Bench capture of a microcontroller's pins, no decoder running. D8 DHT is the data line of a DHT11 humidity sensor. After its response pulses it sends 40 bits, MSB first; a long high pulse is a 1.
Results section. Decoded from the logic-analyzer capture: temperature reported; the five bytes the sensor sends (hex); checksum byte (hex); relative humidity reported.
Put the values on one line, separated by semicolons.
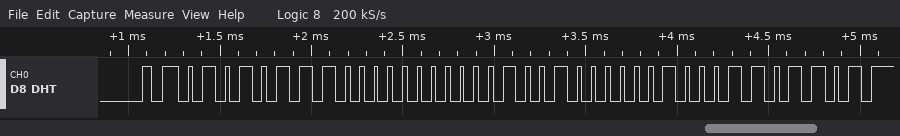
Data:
18.4 °C; 57 00 12 04 6D; 0x6D; 87 %
